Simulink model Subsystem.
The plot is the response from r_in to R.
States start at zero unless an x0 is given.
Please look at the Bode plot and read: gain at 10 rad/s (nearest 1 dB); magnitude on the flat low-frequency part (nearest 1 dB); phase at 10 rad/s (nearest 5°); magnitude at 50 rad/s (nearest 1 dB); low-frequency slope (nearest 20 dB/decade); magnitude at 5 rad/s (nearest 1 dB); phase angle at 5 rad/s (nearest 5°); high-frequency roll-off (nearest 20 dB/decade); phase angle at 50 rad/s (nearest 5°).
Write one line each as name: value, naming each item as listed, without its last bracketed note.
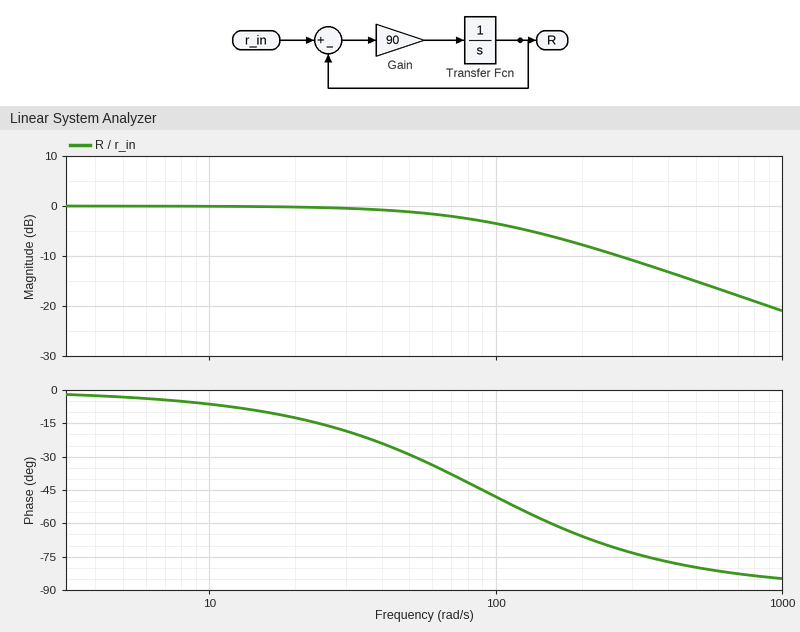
gain at 10 rad/s: 0 dB
magnitude on the flat low-frequency part: 0 dB
phase at 10 rad/s: -5°
magnitude at 50 rad/s: -1 dB
low-frequency slope: 0 dB/decade
magnitude at 5 rad/s: 0 dB
phase angle at 5 rad/s: -5°
high-frequency roll-off: -20 dB/decade
phase angle at 50 rad/s: -30°
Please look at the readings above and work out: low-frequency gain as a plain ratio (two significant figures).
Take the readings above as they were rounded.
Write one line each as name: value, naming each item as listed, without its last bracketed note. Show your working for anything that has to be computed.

low-frequency gain as a plain ratio: 10^(0 / 20) = 1.0
